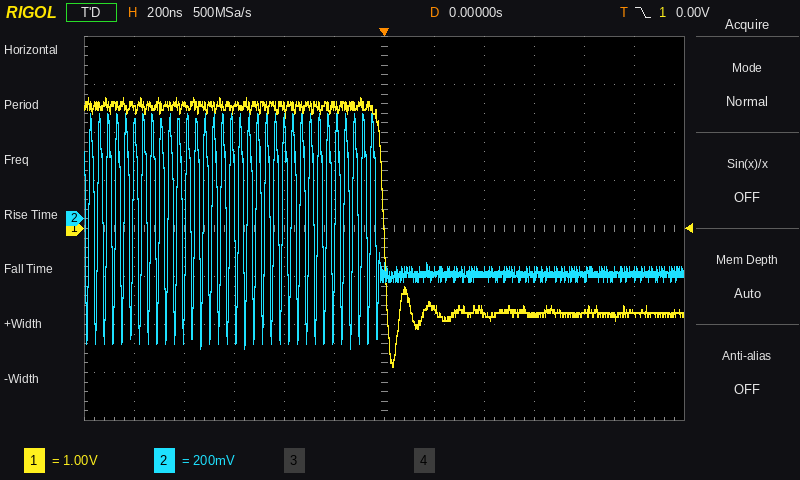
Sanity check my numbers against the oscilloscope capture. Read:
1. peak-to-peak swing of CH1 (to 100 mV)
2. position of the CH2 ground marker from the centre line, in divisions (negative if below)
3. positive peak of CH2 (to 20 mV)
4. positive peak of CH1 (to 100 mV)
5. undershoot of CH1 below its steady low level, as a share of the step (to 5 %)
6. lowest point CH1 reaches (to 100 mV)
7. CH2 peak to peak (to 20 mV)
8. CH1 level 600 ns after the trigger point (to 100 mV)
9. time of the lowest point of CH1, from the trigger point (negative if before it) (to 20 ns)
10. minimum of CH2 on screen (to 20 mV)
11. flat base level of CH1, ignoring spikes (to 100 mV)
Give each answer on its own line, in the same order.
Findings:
5.6 V
+0.2 div
440 mV
2.7 V
25 %
-2.9 V
980 mV
-1.8 V
+40 ns
-540 mV
-1.8 V
